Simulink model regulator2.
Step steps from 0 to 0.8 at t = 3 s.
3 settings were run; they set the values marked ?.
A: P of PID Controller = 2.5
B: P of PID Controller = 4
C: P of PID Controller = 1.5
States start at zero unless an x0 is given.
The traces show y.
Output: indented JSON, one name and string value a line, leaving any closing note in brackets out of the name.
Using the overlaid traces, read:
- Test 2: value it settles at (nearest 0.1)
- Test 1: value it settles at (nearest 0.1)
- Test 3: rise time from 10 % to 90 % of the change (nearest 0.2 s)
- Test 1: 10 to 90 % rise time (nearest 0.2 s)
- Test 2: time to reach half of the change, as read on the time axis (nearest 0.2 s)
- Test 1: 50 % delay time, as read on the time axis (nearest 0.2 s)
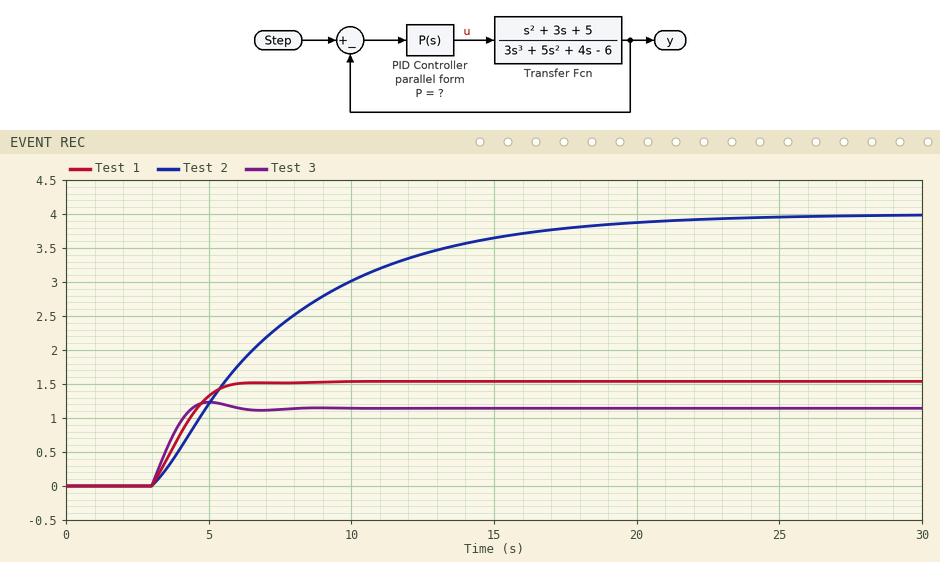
{
  "Test 2: value it settles at": "4.0",
  "Test 1: value it settles at": "1.5",
  "Test 3: rise time from 10 % to 90 % of the change": "1.0 s",
  "Test 1: 10 to 90 % rise time": "2.0 s",
  "Test 2: time to reach half of the change, as read on the time axis": "6.6 s",
  "Test 1: 50 % delay time, as read on the time axis": "4.0 s"
}
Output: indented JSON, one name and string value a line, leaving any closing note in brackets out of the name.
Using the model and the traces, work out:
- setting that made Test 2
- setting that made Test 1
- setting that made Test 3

{
  "setting that made Test 2": "C",
  "setting that made Test 1": "A",
  "setting that made Test 3": "B"
}
